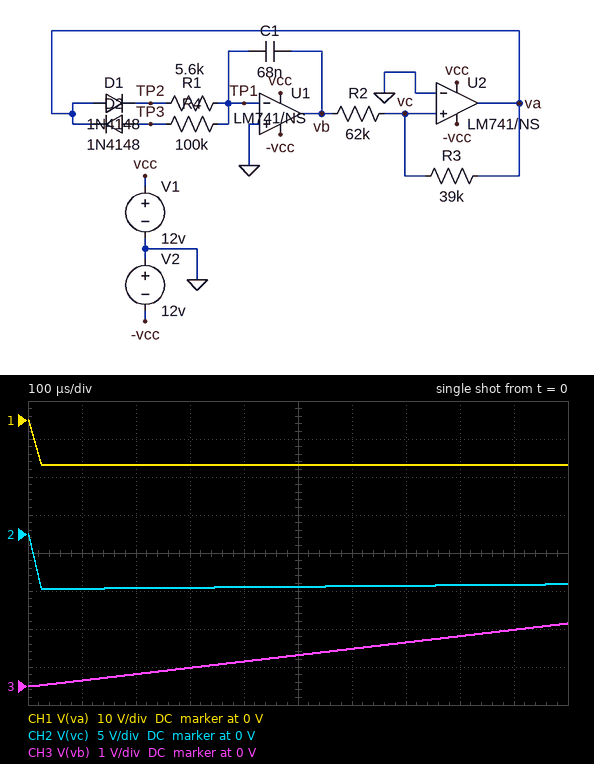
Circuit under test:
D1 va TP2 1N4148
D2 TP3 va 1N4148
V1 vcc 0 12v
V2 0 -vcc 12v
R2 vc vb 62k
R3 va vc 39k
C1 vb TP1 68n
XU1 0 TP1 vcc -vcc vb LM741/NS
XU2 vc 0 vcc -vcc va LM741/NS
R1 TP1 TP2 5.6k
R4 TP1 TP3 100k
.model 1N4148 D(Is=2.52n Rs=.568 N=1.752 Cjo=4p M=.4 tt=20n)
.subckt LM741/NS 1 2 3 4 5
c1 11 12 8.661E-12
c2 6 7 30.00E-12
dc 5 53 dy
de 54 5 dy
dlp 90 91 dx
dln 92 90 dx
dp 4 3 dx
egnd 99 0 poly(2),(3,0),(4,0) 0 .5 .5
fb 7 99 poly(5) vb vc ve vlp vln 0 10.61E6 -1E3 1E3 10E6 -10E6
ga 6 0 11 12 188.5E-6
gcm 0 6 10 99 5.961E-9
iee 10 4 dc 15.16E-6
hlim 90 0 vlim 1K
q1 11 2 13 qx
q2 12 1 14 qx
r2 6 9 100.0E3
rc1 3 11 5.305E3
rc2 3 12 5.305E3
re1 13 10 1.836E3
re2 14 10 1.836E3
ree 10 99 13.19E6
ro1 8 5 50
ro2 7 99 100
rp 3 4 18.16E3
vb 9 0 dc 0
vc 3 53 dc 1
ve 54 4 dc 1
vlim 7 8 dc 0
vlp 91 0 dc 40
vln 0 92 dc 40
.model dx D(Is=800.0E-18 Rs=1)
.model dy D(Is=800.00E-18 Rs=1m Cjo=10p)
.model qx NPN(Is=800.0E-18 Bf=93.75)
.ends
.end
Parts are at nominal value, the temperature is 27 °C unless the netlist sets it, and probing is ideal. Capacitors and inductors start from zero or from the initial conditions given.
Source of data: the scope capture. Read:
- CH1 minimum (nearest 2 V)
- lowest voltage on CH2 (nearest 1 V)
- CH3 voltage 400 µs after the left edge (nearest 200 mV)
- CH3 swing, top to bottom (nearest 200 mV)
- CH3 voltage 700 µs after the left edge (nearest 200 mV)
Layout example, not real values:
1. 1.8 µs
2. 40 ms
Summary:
1. -12 V
2. -7 V
3. 600 mV
4. 1.6 V
5. 1.2 V
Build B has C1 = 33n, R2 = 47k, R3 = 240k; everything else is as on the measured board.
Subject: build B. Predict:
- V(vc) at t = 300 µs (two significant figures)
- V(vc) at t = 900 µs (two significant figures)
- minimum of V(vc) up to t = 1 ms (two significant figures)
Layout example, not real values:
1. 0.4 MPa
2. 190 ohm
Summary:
1. -1.1 V
2. -4.6 V
3. -4.7 V
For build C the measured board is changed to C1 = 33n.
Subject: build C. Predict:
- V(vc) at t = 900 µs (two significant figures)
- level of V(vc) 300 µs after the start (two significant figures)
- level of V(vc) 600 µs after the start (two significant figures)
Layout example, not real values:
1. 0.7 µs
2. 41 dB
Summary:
1. -6.1 V
2. -6.9 V
3. -6.5 V
